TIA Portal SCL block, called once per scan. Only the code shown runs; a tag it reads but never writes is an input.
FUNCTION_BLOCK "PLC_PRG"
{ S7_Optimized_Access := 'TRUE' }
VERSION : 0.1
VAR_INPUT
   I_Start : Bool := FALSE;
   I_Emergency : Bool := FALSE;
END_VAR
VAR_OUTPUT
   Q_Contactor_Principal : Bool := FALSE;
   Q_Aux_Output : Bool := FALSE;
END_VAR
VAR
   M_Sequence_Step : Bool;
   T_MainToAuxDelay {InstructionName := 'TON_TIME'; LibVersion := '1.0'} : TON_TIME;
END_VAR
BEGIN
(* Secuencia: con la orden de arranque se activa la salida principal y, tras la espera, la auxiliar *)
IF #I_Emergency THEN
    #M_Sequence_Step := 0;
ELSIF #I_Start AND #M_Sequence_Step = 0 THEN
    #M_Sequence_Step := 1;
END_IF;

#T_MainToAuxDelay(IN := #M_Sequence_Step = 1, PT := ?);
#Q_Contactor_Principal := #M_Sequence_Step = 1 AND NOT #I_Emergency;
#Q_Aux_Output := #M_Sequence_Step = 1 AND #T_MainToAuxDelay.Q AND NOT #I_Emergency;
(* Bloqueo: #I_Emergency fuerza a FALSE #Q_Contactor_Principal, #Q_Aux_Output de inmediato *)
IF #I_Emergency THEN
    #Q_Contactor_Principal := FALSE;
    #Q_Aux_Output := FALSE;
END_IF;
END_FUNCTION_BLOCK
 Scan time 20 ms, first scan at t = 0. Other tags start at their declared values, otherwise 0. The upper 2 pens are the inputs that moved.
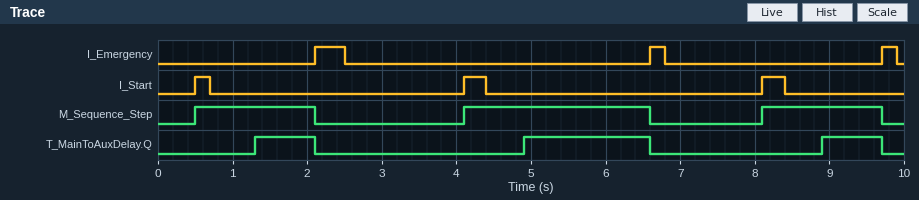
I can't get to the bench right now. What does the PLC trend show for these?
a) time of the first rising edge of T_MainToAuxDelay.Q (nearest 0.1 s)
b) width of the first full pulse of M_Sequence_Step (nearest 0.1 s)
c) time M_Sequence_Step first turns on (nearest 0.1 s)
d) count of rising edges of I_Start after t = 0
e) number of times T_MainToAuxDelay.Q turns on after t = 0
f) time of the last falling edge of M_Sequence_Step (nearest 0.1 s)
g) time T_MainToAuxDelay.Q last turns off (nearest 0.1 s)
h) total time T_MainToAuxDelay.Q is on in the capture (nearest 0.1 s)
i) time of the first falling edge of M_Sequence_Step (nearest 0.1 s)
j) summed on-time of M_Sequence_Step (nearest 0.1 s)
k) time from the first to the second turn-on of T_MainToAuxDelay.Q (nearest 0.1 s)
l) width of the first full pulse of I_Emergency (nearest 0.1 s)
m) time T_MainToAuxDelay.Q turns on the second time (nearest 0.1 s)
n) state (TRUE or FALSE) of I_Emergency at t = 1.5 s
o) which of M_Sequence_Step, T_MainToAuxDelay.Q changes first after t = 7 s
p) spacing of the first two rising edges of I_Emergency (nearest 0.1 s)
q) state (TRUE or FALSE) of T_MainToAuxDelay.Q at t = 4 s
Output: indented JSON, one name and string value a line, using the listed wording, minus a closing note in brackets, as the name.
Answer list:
{
  "time of the first rising edge of T_MainToAuxDelay.Q": "1.3 s",
  "width of the first full pulse of M_Sequence_Step": "1.6 s",
  "time M_Sequence_Step first turns on": "0.5 s",
  "count of rising edges of I_Start after t = 0": "3",
  "number of times T_MainToAuxDelay.Q turns on after t = 0": "3",
  "time of the last falling edge of M_Sequence_Step": "9.7 s",
  "time T_MainToAuxDelay.Q last turns off": "9.7 s",
  "total time T_MainToAuxDelay.Q is on in the capture": "3.3 s",
  "time of the first falling edge of M_Sequence_Step": "2.1 s",
  "summed on-time of M_Sequence_Step": "5.7 s",
  "time from the first to the second turn-on of T_MainToAuxDelay.Q": "3.6 s",
  "width of the first full pulse of I_Emergency": "0.4 s",
  "time T_MainToAuxDelay.Q turns on the second time": "4.9 s",
  "state (TRUE or FALSE) of I_Emergency at t = 1.5 s": "FALSE",
  "which of M_Sequence_Step, T_MainToAuxDelay.Q changes first after t = 7 s": "M_Sequence_Step",
  "spacing of the first two rising edges of I_Emergency": "4.5 s",
  "state (TRUE or FALSE) of T_MainToAuxDelay.Q at t = 4 s": "FALSE"
}
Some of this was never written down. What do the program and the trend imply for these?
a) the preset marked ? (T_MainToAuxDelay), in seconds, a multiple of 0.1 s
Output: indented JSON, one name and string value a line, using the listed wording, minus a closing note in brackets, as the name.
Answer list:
{
  "the preset marked ? (T_MainToAuxDelay), in seconds, a multiple of 0.1 s": "0.8 s"
}
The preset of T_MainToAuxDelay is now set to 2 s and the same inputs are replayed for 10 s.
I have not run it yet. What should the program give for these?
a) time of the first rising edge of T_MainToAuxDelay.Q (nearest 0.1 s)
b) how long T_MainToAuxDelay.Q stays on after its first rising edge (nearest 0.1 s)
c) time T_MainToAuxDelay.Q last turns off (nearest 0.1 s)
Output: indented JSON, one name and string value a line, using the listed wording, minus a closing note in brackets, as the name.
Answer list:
{
  "time of the first rising edge of T_MainToAuxDelay.Q": "6.1 s",
  "how long T_MainToAuxDelay.Q stays on after its first rising edge": "0.5 s",
  "time T_MainToAuxDelay.Q last turns off": "6.6 s"
}
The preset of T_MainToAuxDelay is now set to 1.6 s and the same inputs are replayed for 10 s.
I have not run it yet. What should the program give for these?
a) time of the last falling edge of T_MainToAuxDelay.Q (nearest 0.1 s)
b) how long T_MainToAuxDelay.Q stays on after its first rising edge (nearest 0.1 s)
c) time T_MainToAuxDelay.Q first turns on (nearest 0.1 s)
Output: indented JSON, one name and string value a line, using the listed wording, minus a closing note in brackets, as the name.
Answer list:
{
  "time of the last falling edge of T_MainToAuxDelay.Q": "6.6 s",
  "how long T_MainToAuxDelay.Q stays on after its first rising edge": "0.9 s",
  "time T_MainToAuxDelay.Q first turns on": "5.7 s"
}
